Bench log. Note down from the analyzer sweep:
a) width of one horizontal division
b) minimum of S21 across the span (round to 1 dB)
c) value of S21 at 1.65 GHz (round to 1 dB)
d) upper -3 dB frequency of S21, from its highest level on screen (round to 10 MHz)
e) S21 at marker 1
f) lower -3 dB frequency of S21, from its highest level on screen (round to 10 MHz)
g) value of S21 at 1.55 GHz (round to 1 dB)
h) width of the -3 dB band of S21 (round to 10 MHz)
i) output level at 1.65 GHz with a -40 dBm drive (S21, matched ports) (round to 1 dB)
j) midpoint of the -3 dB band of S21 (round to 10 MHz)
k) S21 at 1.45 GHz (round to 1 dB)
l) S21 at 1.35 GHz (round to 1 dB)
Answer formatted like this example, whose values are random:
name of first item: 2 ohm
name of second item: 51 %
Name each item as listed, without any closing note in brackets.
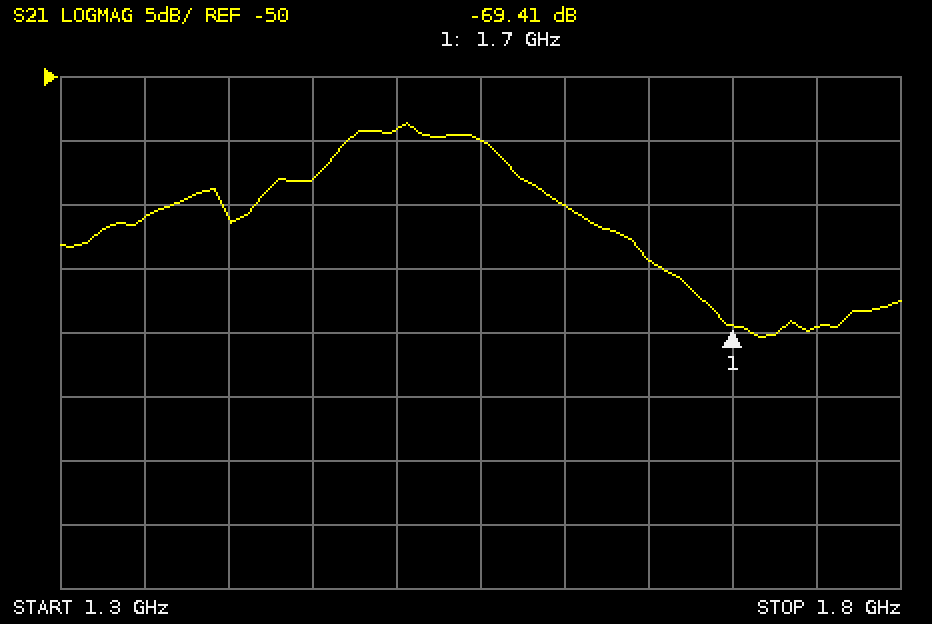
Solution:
width of one horizontal division: 50 MHz
minimum of S21 across the span: -70 dB
value of S21 at 1.65 GHz: -64 dB
upper -3 dB frequency of S21, from its highest level on screen: 1.56 GHz
S21 at marker 1: -69.41 dB
lower -3 dB frequency of S21, from its highest level on screen: 1.46 GHz
value of S21 at 1.55 GHz: -55 dB
width of the -3 dB band of S21: 100 MHz
output level at 1.65 GHz with a -40 dBm drive (S21, matched ports): -104 dBm
midpoint of the -3 dB band of S21: 1.51 GHz
S21 at 1.45 GHz: -58 dB
S21 at 1.35 GHz: -61 dB
